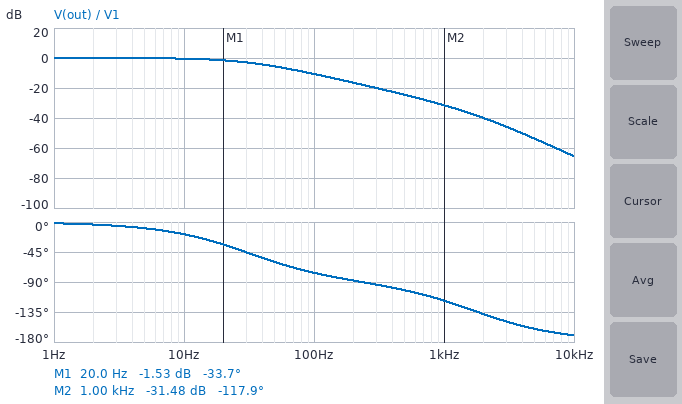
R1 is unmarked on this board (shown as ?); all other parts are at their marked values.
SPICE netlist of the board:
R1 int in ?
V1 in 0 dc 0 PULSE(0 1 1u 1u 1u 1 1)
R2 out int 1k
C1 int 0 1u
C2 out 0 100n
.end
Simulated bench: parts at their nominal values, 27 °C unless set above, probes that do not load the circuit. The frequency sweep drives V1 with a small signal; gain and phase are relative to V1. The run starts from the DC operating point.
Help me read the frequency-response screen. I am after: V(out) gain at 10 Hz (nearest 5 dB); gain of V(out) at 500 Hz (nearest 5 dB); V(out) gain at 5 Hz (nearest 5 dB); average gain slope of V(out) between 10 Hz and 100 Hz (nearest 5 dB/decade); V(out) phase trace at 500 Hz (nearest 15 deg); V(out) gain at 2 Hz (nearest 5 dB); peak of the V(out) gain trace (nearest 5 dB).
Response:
0 dB
-25 dB
0 dB
-10 dB/decade
-105 deg
0 dB
0 dB
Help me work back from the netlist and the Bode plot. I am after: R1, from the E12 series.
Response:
4.7 kΩ
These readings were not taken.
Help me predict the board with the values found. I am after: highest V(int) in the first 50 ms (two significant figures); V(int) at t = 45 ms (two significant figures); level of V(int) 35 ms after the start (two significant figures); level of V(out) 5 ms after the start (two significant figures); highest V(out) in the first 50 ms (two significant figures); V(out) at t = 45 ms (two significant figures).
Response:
1.0 V
1.0 V
1.0 V
610 mV
1.0 V
1.0 V
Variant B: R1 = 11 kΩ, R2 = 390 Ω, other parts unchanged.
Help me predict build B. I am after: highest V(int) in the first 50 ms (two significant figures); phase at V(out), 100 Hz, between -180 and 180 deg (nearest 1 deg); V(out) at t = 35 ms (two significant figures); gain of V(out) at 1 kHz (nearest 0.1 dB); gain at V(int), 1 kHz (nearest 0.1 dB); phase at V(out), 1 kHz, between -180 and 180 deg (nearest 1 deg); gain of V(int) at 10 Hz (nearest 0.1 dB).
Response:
980 mV
-84 deg
940 mV
-37.8 dB
-37.6 dB
-102 deg
-2.0 dB
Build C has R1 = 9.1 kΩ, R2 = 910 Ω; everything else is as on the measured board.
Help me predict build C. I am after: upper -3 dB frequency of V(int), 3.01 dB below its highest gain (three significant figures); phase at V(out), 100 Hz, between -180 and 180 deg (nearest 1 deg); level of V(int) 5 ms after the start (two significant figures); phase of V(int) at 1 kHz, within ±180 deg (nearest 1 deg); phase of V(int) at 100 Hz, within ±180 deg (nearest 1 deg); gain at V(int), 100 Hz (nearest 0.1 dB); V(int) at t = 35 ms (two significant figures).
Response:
15.9 Hz
-84 deg
390 mV
-87 deg
-81 deg
-16.1 dB
970 mV
